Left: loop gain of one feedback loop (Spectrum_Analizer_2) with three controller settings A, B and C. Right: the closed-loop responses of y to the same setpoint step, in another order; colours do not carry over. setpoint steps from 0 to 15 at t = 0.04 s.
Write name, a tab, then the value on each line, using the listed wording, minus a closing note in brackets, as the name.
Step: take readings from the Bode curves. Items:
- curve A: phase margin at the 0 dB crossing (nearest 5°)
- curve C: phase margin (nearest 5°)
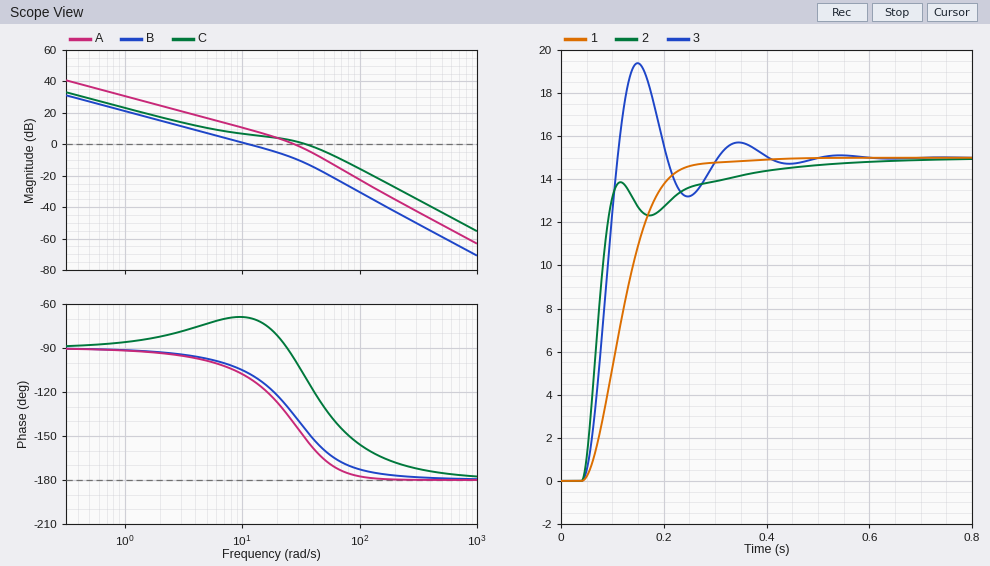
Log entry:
curve A: phase margin at the 0 dB crossing	40°
curve C: phase margin	70°
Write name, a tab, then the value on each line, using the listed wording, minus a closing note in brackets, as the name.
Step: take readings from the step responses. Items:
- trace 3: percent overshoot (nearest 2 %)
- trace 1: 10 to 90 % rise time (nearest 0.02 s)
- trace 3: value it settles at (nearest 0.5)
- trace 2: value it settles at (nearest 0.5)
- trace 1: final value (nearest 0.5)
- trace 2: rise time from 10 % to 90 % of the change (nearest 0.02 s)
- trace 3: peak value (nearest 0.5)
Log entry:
trace 3: percent overshoot	30 %
trace 1: 10 to 90 % rise time	0.12 s
trace 3: value it settles at	15.0
trace 2: value it settles at	15.0
trace 1: final value	15.0
trace 2: rise time from 10 % to 90 % of the change	0.06 s
trace 3: peak value	19.5
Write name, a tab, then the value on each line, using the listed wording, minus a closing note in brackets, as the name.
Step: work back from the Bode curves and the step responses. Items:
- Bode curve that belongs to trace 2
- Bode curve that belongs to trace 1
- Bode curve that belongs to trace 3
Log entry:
Bode curve that belongs to trace 2	C
Bode curve that belongs to trace 1	B
Bode curve that belongs to trace 3	A
